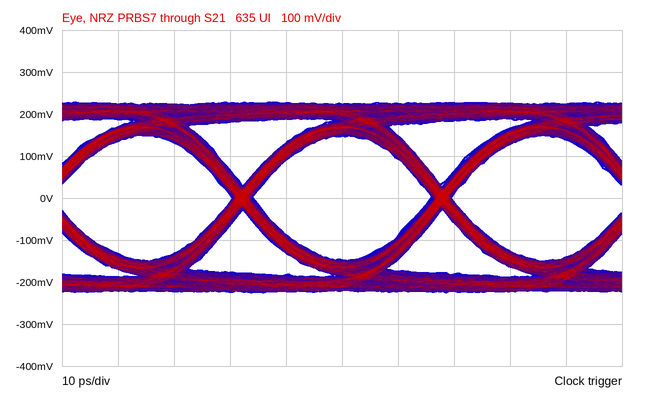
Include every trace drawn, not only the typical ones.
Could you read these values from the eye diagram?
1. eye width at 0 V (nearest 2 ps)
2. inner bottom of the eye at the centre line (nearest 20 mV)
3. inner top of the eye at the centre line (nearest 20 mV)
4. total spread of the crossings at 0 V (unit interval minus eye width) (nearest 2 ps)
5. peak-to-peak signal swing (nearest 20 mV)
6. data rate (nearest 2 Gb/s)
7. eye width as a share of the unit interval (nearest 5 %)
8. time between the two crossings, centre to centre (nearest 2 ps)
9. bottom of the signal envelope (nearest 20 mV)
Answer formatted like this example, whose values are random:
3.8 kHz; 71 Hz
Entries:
32 ps; -140 mV; 140 mV; 4 ps; 460 mV; 28 Gb/s; 90 %; 36 ps; -220 mV
